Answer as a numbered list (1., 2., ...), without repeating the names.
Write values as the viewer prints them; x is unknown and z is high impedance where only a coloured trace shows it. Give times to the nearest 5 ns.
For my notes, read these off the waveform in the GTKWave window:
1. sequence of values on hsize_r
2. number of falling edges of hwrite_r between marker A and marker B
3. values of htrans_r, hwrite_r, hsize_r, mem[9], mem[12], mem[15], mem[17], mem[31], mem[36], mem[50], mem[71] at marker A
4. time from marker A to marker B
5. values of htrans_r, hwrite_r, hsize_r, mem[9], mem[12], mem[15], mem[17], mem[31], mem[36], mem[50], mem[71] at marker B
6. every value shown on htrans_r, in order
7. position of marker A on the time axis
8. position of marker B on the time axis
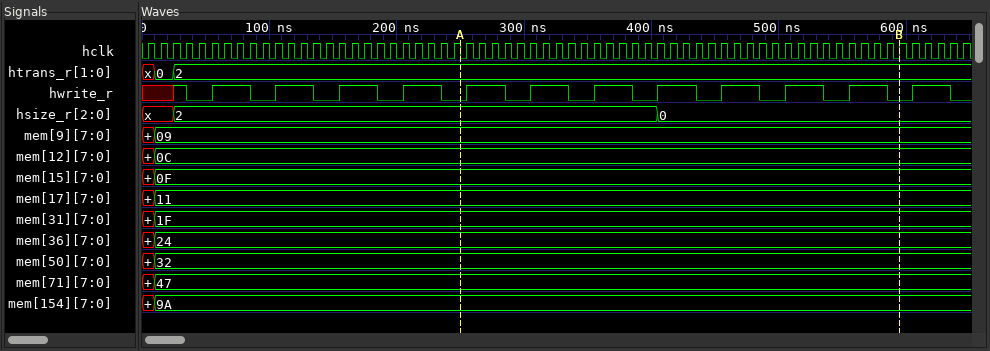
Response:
1. x, 2, 0
2. 7
3. htrans_r=2, hwrite_r=0, hsize_r=2, mem[9]=09, mem[12]=0C, mem[15]=0F, mem[17]=11, mem[31]=1F, mem[36]=24, mem[50]=32, mem[71]=47
4. 345 ns
5. htrans_r=2, hwrite_r=0, hsize_r=0, mem[9]=09, mem[12]=0C, mem[15]=0F, mem[17]=11, mem[31]=1F, mem[36]=24, mem[50]=32, mem[71]=47
6. x, 0, 2
7. 250 ns
8. 595 ns
